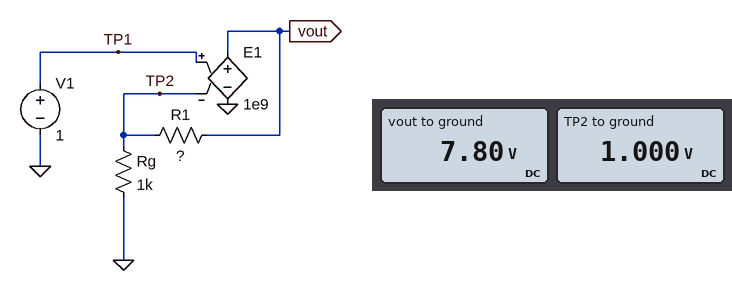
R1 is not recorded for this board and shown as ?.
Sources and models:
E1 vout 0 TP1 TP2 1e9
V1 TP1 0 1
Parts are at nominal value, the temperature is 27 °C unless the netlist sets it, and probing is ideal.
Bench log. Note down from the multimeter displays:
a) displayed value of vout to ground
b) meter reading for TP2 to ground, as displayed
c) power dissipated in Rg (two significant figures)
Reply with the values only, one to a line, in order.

7.80 V
1.000 V
1.0 mW
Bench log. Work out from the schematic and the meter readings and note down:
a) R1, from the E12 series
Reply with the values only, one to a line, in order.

6.8 kΩ
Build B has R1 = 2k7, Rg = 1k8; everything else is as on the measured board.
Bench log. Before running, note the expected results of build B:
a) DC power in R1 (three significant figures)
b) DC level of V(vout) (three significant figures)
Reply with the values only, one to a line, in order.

833 µW
2.50 V
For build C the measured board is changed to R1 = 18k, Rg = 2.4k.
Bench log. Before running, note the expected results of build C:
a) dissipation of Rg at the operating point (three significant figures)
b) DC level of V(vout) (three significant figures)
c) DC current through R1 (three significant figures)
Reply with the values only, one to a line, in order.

417 µW
8.50 V
417 µA
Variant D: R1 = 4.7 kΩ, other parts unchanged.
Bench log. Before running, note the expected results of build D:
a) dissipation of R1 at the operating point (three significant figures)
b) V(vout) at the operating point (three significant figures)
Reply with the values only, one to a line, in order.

4.70 mW
5.70 V
